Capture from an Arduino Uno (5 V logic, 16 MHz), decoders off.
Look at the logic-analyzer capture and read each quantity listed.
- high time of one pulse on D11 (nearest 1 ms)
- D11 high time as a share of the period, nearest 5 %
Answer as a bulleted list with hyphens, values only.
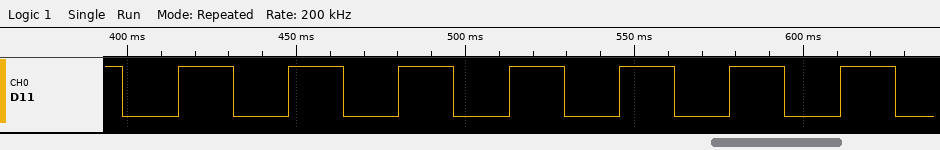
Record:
- 16 ms
- 50 %
